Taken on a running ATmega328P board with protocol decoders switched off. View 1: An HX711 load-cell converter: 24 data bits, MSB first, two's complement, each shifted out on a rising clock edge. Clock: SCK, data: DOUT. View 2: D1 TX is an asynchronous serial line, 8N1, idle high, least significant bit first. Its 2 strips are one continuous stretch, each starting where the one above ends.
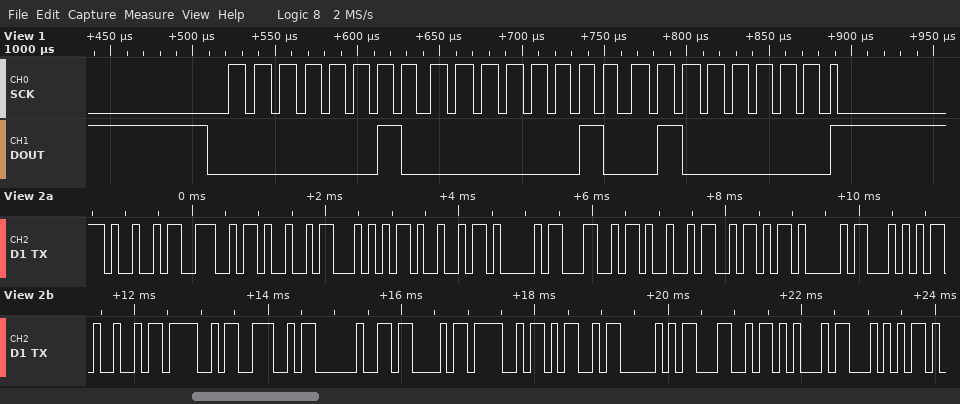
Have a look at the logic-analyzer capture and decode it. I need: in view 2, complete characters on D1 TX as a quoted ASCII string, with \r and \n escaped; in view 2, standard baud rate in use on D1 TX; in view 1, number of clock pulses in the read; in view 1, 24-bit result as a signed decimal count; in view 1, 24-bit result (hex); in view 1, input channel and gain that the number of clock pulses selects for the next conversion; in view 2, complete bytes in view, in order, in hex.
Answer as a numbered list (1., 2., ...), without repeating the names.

1. "INITIALIZATION COMPLET"
2. 9600 baud
3. 25
4. 131648
5. 0x020240
6. channel A, gain 128
7. 0x49 0x4E 0x49 0x54 0x49 0x41 0x4C 0x49 0x5A 0x41 0x54 0x49 0x4F 0x4E 0x20 0x43 0x4F 0x4D 0x50 0x4C 0x45 0x54
